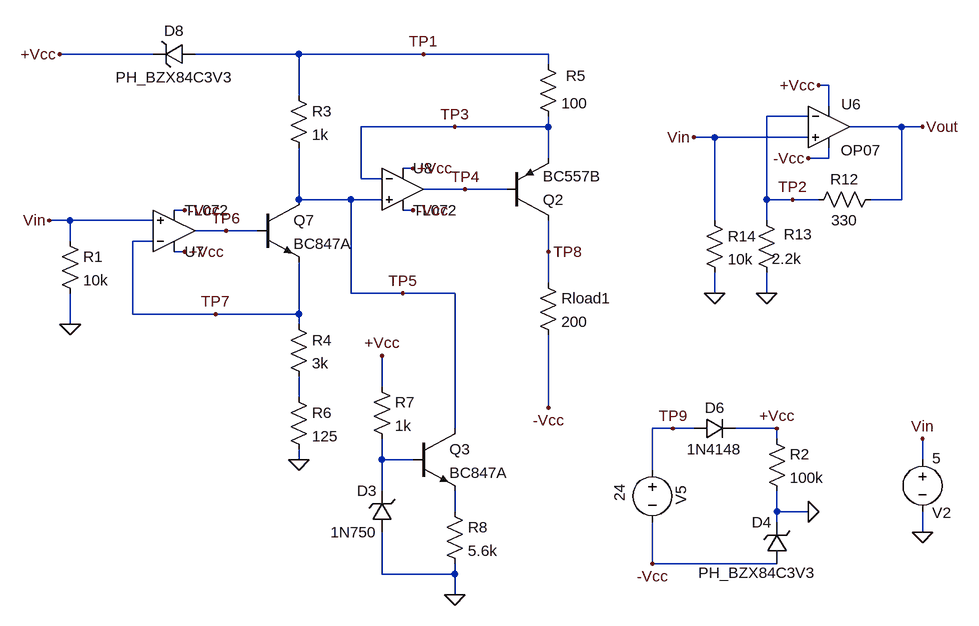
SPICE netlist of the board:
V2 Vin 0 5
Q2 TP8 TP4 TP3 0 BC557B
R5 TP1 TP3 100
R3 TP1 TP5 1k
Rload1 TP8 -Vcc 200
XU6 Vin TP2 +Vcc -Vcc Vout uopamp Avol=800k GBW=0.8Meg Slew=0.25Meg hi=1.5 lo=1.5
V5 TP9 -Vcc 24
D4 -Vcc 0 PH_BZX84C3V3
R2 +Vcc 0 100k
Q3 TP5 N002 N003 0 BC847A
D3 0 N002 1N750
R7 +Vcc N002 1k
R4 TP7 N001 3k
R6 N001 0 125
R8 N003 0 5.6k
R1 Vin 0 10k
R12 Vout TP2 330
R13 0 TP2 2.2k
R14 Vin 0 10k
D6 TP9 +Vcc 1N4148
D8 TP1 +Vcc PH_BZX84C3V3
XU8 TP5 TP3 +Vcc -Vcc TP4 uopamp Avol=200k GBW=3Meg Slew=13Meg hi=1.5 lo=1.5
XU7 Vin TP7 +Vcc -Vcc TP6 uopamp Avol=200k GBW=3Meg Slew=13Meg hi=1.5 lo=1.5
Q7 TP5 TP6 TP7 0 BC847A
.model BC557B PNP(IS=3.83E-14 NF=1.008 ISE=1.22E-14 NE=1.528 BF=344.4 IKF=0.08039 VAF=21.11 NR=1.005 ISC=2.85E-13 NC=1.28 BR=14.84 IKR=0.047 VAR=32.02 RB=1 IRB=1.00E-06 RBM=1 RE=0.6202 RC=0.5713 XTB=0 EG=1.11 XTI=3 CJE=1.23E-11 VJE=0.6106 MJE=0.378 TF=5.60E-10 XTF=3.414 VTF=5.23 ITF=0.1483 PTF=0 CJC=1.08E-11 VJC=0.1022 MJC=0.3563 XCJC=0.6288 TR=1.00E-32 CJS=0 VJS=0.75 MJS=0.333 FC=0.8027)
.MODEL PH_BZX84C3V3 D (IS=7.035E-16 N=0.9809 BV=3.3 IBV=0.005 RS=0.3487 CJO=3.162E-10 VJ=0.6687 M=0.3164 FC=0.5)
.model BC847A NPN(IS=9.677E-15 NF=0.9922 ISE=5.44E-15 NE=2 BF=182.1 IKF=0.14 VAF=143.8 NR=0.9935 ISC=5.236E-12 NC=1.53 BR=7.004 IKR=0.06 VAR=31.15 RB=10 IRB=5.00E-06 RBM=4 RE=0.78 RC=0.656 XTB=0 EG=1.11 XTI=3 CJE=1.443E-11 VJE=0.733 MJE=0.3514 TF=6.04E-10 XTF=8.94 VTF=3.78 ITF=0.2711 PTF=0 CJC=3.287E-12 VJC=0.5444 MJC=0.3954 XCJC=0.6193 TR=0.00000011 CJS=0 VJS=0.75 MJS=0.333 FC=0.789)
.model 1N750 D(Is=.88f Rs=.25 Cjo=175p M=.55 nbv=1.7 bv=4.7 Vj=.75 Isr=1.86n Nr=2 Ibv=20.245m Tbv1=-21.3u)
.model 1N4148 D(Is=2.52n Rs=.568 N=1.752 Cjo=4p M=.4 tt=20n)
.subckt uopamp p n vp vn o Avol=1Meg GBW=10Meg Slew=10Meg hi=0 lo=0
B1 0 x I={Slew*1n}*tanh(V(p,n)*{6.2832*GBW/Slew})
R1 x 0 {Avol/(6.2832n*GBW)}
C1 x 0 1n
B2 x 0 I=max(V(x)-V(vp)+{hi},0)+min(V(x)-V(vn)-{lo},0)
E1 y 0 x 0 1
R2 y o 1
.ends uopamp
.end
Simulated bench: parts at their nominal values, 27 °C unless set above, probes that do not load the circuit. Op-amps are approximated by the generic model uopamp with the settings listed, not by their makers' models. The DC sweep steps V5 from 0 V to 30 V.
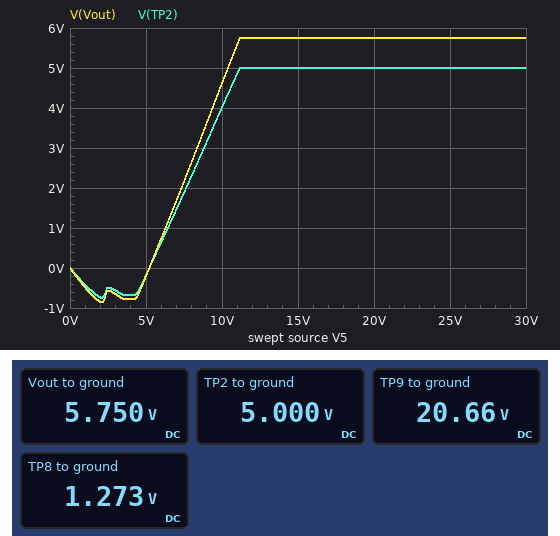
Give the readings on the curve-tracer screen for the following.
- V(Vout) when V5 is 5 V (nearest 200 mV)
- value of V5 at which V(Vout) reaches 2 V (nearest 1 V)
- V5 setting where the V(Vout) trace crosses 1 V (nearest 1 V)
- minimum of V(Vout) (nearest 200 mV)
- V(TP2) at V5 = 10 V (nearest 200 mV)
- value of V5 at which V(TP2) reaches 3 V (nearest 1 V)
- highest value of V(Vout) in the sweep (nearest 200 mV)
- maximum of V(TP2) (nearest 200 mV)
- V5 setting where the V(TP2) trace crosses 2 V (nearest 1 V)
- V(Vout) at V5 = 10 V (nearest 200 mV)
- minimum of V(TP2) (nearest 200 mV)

-200 mV
7 V
6 V
-800 mV
4.0 V
9 V
5.8 V
5.0 V
8 V
4.6 V
-800 mV
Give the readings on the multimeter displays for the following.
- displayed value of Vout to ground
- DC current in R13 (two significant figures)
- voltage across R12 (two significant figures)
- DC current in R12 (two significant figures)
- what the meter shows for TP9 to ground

5.750 V
2.3 mA
750 mV
2.3 mA
20.66 V
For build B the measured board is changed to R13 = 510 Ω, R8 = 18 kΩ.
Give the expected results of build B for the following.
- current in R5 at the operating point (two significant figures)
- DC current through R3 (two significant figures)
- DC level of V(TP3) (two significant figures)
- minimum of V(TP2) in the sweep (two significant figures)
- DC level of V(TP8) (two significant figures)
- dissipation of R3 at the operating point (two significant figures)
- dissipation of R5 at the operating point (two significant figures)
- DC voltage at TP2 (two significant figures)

18 mA
1.8 mA
15 V
-520 mV
290 mV
3.3 mW
33 mW
5.0 V
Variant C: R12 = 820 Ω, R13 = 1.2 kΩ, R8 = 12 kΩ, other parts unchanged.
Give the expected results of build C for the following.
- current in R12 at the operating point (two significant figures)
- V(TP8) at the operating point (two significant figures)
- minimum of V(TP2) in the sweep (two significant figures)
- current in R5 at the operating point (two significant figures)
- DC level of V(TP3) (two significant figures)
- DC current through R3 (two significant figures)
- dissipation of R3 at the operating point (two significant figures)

4.2 mA
510 mV
-510 mV
19 mA
15 V
1.9 mA
3.7 mW
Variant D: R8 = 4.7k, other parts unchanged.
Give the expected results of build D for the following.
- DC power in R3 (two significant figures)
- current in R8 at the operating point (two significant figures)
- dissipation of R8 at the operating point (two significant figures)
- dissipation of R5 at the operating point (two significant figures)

6.0 mW
860 µA
3.5 mW
60 mW
